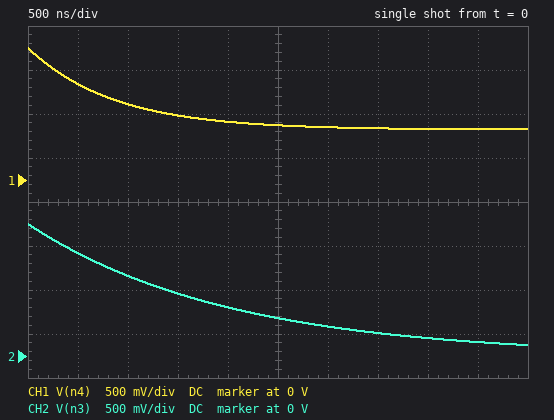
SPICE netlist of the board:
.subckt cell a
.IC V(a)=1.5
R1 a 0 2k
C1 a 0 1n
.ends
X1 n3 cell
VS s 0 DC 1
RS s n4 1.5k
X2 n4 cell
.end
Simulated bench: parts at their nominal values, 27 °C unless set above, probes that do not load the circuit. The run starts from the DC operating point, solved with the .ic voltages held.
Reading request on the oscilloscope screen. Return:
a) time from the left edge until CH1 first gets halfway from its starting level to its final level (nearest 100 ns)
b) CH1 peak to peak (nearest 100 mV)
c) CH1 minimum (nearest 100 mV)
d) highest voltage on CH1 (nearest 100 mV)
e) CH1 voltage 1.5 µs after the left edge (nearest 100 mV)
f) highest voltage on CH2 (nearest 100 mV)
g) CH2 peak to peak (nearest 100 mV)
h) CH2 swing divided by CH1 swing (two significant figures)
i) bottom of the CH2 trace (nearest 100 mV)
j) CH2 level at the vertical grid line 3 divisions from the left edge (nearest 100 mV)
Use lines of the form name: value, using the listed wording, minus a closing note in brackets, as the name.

time from the left edge until CH1 first gets halfway from its starting level to its final level: 600 ns
CH1 peak to peak: 900 mV
CH1 minimum: 600 mV
highest voltage on CH1: 1.5 V
CH1 voltage 1.5 µs after the left edge: 700 mV
highest voltage on CH2: 1.5 V
CH2 peak to peak: 1.4 V
CH2 swing divided by CH1 swing: 1.5
bottom of the CH2 trace: 100 mV
CH2 level at the vertical grid line 3 divisions from the left edge: 700 mV
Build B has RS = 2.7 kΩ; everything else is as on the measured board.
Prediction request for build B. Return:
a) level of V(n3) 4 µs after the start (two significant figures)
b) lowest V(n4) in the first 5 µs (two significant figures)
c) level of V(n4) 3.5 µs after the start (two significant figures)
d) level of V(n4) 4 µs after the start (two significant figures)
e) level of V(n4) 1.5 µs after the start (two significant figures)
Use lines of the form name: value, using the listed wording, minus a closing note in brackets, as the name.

level of V(n3) 4 µs after the start: 200 mV
lowest V(n4) in the first 5 µs: 440 mV
level of V(n4) 3.5 µs after the start: 480 mV
level of V(n4) 4 µs after the start: 460 mV
level of V(n4) 1.5 µs after the start: 720 mV
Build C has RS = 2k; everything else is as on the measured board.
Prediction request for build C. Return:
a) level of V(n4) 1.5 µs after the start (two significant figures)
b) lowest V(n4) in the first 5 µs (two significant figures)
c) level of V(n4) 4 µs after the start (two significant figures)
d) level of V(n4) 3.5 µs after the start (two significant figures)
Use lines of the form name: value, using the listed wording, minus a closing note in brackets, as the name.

level of V(n4) 1.5 µs after the start: 720 mV
lowest V(n4) in the first 5 µs: 510 mV
level of V(n4) 4 µs after the start: 520 mV
level of V(n4) 3.5 µs after the start: 530 mV
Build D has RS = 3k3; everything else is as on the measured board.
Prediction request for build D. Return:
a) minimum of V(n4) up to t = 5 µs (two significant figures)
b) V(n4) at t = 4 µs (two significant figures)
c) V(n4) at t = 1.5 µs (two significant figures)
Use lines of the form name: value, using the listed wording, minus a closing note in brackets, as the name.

minimum of V(n4) up to t = 5 µs: 400 mV
V(n4) at t = 4 µs: 420 mV
V(n4) at t = 1.5 µs: 710 mV
